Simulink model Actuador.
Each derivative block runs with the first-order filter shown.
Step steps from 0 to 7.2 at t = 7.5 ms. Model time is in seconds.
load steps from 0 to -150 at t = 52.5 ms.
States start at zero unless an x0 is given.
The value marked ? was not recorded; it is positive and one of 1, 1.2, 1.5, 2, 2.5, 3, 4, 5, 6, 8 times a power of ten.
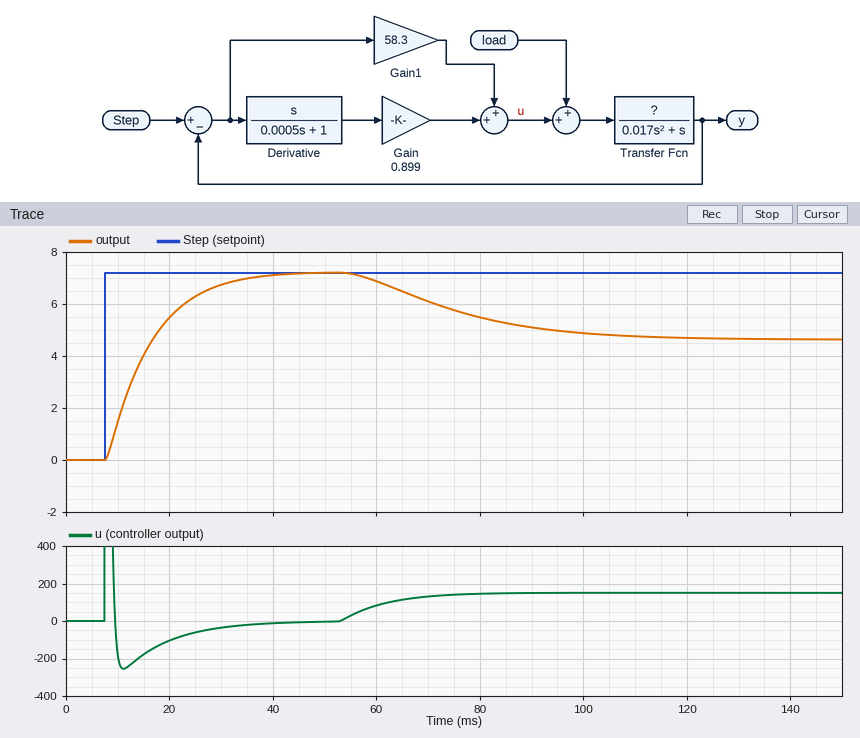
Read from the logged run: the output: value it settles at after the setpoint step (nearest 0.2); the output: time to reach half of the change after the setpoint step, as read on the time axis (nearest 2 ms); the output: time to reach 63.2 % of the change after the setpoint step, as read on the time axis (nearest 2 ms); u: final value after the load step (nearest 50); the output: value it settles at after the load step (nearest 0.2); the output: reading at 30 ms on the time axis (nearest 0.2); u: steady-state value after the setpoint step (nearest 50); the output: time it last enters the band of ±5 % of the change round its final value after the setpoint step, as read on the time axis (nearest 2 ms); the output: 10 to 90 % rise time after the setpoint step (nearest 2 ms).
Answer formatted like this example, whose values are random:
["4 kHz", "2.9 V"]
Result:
["7.2", "14 ms", "16 ms", "150", "4.6", "6.8", "0", "32 ms", "18 ms"]
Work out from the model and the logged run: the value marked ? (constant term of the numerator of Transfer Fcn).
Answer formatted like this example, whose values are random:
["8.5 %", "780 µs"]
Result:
["2"]
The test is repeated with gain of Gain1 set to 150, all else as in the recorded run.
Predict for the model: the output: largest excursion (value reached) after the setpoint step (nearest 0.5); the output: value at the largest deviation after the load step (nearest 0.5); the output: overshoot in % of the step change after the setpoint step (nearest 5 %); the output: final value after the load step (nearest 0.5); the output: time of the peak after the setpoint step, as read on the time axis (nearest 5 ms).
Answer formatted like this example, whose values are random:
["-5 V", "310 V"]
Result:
["8.0", "6.0", "15 %", "6.0", "30 ms"]
